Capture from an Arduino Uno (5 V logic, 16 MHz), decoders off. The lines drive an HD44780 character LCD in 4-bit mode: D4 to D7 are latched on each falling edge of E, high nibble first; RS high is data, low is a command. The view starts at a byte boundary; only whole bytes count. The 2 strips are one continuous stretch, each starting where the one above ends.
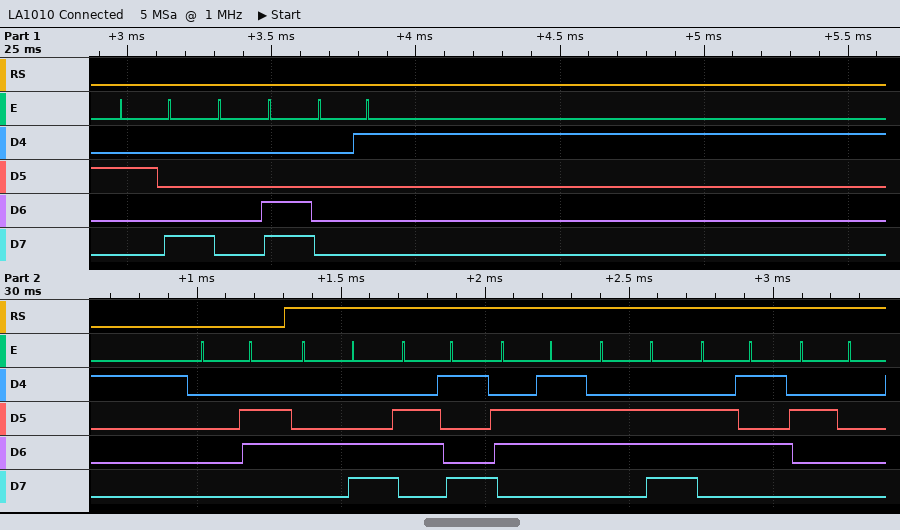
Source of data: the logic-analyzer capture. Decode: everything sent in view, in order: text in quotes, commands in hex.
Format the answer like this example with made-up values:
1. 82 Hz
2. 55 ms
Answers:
1. 0x28 0x0C 0x01 0x06 "Ligne "
